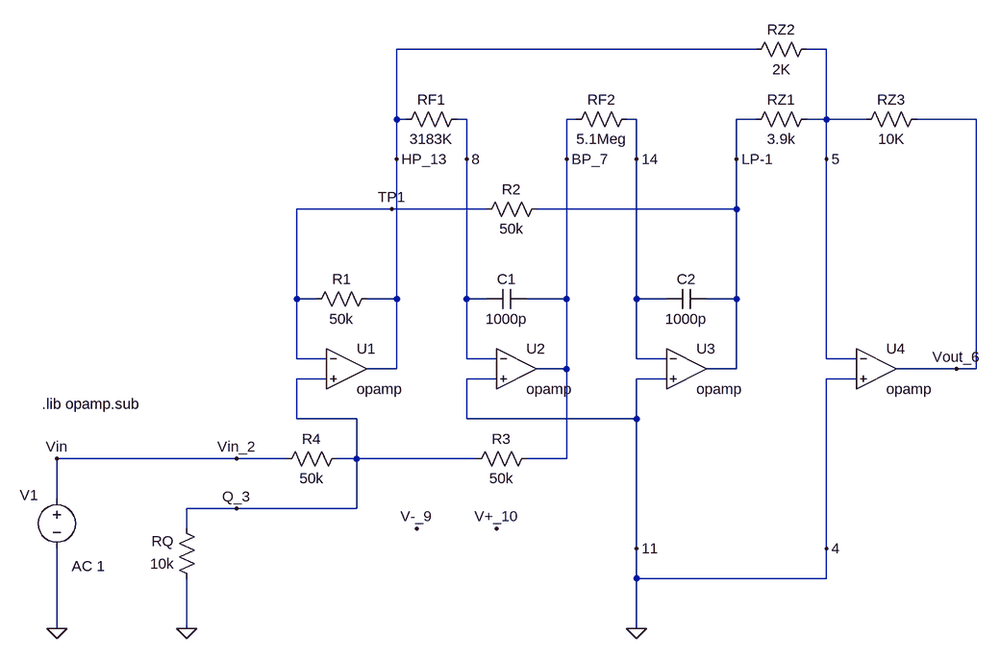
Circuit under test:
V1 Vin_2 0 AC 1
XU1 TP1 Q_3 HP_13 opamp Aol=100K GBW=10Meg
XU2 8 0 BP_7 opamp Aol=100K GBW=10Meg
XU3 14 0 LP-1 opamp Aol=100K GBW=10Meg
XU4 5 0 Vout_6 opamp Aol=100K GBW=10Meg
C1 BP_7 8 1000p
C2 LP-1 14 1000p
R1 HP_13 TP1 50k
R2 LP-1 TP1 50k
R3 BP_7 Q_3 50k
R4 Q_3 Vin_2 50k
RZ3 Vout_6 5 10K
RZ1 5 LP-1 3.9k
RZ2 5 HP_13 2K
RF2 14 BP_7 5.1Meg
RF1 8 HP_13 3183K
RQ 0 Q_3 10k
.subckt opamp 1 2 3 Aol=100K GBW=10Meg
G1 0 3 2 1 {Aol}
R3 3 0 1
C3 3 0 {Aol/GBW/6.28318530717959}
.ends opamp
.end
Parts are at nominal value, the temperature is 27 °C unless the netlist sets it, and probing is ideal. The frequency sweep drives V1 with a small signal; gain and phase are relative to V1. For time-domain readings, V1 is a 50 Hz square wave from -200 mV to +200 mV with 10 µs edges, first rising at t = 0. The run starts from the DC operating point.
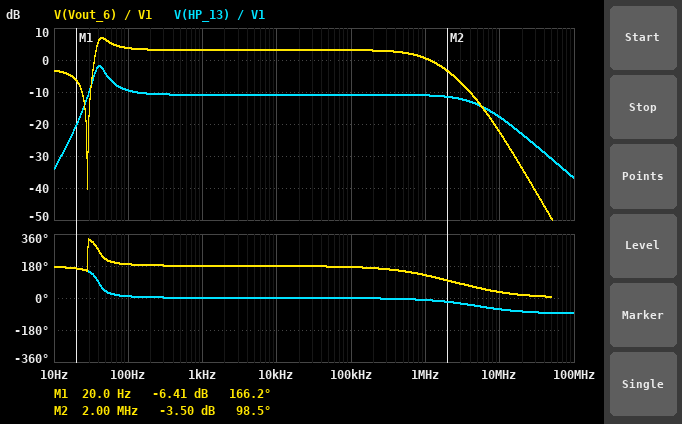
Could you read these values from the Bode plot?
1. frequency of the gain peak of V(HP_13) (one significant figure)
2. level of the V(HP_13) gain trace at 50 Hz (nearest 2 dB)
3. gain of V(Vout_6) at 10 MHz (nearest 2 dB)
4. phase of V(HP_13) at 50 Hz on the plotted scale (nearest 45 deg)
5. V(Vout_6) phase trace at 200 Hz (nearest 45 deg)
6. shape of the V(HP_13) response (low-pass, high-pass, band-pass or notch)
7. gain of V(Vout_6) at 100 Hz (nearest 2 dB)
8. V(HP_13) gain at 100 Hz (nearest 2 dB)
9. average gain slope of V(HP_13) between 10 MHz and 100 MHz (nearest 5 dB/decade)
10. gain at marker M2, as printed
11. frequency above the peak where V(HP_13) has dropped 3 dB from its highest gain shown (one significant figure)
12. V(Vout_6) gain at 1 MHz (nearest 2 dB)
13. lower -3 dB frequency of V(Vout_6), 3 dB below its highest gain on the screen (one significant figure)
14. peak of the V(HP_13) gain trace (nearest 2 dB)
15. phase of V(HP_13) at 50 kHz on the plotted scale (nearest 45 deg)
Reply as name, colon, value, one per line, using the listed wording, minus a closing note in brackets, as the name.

frequency of the gain peak of V(HP_13): 40 Hz
level of the V(HP_13) gain trace at 50 Hz: -4 dB
gain of V(Vout_6) at 10 MHz: -22 dB
phase of V(HP_13) at 50 Hz on the plotted scale: 45 deg
V(Vout_6) phase trace at 200 Hz: 180 deg
shape of the V(HP_13) response: band-pass
gain of V(Vout_6) at 100 Hz: 4 dB
V(HP_13) gain at 100 Hz: -10 dB
average gain slope of V(HP_13) between 10 MHz and 100 MHz: -20 dB/decade
gain at marker M2, as printed: -3.50 dB
frequency above the peak where V(HP_13) has dropped 3 dB from its highest gain shown: 50 Hz
V(Vout_6) gain at 1 MHz: 0 dB
lower -3 dB frequency of V(Vout_6), 3 dB below its highest gain on the screen: 40 Hz
peak of the V(HP_13) gain trace: -2 dB
phase of V(HP_13) at 50 kHz on the plotted scale: 0 deg
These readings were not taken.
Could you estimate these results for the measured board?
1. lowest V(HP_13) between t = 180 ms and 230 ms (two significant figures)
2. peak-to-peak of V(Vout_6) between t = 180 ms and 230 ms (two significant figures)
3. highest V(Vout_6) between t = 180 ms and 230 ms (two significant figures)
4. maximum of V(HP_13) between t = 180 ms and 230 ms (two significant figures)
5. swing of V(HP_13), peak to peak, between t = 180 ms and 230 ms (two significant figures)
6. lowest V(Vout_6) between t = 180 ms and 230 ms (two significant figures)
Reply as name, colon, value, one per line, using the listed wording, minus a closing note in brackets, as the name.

lowest V(HP_13) between t = 180 ms and 230 ms: -160 mV
peak-to-peak of V(Vout_6) between t = 180 ms and 230 ms: 1.3 V
highest V(Vout_6) between t = 180 ms and 230 ms: 630 mV
maximum of V(HP_13) between t = 180 ms and 230 ms: 160 mV
swing of V(HP_13), peak to peak, between t = 180 ms and 230 ms: 330 mV
lowest V(Vout_6) between t = 180 ms and 230 ms: -630 mV
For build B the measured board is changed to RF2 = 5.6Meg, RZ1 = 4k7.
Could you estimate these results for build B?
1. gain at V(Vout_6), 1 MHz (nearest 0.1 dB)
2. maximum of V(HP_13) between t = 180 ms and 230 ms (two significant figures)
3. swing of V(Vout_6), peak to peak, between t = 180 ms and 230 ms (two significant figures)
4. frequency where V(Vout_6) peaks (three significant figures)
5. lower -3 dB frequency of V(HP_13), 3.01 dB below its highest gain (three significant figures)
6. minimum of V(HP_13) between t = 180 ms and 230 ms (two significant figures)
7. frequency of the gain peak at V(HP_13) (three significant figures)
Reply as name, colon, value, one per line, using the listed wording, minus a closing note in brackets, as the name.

gain at V(Vout_6), 1 MHz: 0.7 dB
maximum of V(HP_13) between t = 180 ms and 230 ms: 150 mV
swing of V(Vout_6), peak to peak, between t = 180 ms and 230 ms: 1.2 V
frequency where V(Vout_6) peaks: 41.4 Hz
lower -3 dB frequency of V(HP_13), 3.01 dB below its highest gain: 33.1 Hz
minimum of V(HP_13) between t = 180 ms and 230 ms: -150 mV
frequency of the gain peak at V(HP_13): 39.1 Hz
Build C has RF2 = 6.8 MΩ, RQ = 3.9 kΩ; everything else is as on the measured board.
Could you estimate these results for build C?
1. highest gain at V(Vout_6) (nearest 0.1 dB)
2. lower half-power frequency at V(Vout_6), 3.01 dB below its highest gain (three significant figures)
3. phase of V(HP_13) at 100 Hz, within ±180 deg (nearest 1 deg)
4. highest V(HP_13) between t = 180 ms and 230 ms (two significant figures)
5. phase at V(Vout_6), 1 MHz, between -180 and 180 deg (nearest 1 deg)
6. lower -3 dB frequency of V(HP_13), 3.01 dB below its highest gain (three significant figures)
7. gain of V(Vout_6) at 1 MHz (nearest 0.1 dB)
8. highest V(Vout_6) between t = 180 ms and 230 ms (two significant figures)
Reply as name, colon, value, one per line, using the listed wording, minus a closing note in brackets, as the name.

highest gain at V(Vout_6): 4.8 dB
lower half-power frequency at V(Vout_6), 3.01 dB below its highest gain: 32.5 Hz
phase of V(HP_13) at 100 Hz, within ±180 deg: 4 deg
highest V(HP_13) between t = 180 ms and 230 ms: 57 mV
phase at V(Vout_6), 1 MHz, between -180 and 180 deg: 128 deg
lower -3 dB frequency of V(HP_13), 3.01 dB below its highest gain: 31.5 Hz
gain of V(Vout_6) at 1 MHz: -6.0 dB
highest V(Vout_6) between t = 180 ms and 230 ms: 220 mV
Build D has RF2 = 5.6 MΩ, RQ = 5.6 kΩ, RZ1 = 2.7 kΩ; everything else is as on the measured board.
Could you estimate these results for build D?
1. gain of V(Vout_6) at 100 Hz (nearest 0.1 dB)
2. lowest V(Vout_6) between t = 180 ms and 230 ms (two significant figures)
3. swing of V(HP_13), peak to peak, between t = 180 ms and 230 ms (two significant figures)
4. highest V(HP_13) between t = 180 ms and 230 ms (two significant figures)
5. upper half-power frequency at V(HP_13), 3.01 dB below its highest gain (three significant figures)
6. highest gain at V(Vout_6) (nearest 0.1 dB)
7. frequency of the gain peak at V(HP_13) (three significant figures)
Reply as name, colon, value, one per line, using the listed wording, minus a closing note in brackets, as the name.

gain of V(Vout_6) at 100 Hz: -0.5 dB
lowest V(Vout_6) between t = 180 ms and 230 ms: -310 mV
swing of V(HP_13), peak to peak, between t = 180 ms and 230 ms: 190 mV
highest V(HP_13) between t = 180 ms and 230 ms: 96 mV
upper half-power frequency at V(HP_13), 3.01 dB below its highest gain: 44.1 Hz
highest gain at V(Vout_6): 2.0 dB
frequency of the gain peak at V(HP_13): 38.3 Hz
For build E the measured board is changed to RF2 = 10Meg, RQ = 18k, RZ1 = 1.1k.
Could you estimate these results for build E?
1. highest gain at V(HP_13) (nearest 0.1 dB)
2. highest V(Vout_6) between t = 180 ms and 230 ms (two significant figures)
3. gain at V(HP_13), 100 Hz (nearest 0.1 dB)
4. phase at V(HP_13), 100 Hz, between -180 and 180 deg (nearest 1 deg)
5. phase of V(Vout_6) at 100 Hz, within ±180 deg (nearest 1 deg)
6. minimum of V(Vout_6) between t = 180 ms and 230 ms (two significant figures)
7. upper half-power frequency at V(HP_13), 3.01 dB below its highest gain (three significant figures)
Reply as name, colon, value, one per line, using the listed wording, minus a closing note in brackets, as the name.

highest gain at V(HP_13): -4.3 dB
highest V(Vout_6) between t = 180 ms and 230 ms: 620 mV
gain at V(HP_13), 100 Hz: -7.1 dB
phase at V(HP_13), 100 Hz, between -180 and 180 deg: 13 deg
phase of V(Vout_6) at 100 Hz, within ±180 deg: -167 deg
minimum of V(Vout_6) between t = 180 ms and 230 ms: -620 mV
upper half-power frequency at V(HP_13), 3.01 dB below its highest gain: 149 Hz
